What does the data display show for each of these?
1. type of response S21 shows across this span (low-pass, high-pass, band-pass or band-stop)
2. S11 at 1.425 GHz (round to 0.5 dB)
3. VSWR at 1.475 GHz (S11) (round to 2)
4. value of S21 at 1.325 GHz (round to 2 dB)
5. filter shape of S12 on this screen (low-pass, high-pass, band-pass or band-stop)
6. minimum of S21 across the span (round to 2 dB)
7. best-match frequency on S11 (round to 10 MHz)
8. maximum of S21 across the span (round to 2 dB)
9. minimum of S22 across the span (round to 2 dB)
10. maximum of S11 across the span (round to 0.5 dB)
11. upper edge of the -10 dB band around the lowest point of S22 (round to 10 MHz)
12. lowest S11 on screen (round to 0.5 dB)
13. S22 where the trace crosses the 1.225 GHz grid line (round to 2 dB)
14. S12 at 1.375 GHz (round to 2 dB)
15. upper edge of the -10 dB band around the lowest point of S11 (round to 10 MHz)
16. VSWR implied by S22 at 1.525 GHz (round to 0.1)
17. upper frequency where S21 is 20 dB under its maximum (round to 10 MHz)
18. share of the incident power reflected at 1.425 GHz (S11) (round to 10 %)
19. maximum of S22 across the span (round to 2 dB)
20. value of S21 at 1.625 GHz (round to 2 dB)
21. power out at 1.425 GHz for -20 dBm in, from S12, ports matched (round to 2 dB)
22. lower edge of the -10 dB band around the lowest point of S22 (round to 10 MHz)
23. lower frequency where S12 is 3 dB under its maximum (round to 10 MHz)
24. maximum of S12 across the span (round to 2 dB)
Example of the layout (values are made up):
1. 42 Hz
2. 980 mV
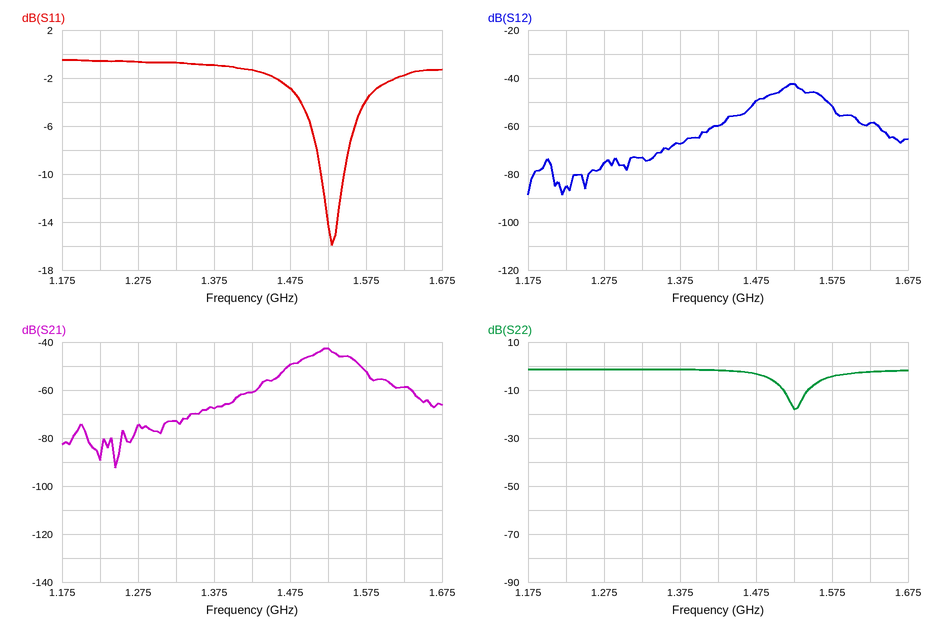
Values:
1. band-pass
2. -1.5 dB
3. 6
4. -72 dB
5. band-pass
6. -92 dB
7. 1.53 GHz
8. -42 dB
9. -18 dB
10. -0.5 dB
11. 1.54 GHz
12. -16.0 dB
13. -2 dB
14. -68 dB
15. 1.55 GHz
16. 1.3
17. 1.64 GHz
18. 70 %
19. -2 dB
20. -58 dB
21. -80 dBm
22. 1.51 GHz
23. 1.51 GHz
24. -42 dB
